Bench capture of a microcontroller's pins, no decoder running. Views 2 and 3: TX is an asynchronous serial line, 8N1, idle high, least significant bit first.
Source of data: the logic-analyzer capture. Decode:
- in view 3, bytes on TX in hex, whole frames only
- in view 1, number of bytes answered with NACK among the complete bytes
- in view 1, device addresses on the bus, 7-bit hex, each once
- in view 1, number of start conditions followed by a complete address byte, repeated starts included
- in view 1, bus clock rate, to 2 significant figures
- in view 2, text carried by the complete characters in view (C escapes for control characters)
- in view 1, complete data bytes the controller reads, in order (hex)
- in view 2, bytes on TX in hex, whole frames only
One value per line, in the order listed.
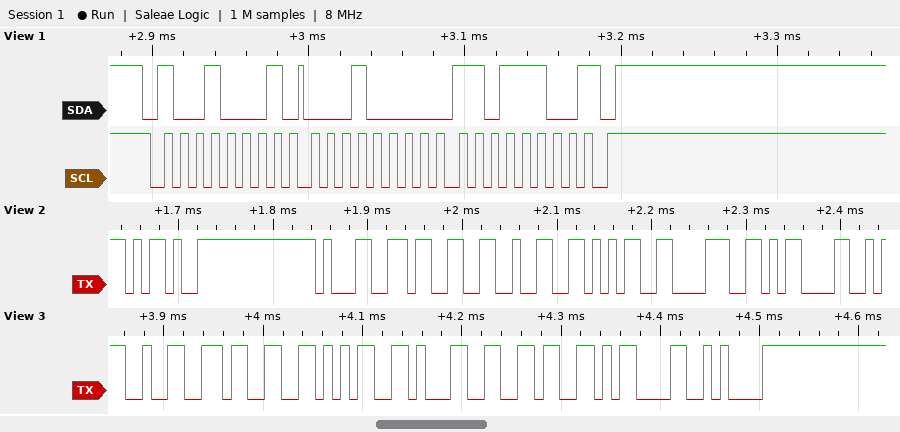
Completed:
0x32 0x33 0x35 0x31 0x36 0x0D 0x0A
1
0x48
1
100 kHz
"-13258\r"
10 DC
0x2D 0x31 0x33 0x32 0x35 0x38 0x0D
